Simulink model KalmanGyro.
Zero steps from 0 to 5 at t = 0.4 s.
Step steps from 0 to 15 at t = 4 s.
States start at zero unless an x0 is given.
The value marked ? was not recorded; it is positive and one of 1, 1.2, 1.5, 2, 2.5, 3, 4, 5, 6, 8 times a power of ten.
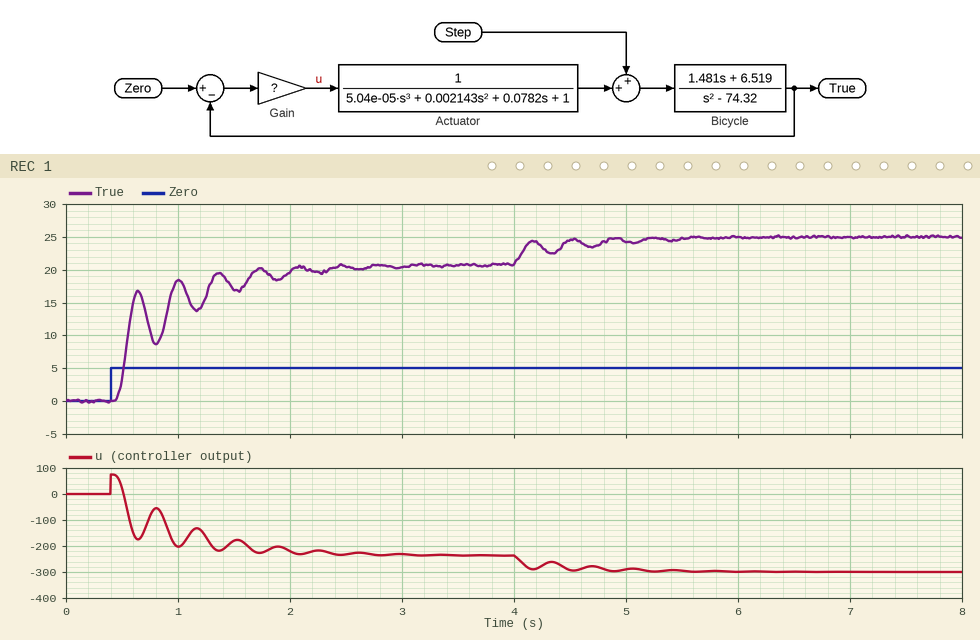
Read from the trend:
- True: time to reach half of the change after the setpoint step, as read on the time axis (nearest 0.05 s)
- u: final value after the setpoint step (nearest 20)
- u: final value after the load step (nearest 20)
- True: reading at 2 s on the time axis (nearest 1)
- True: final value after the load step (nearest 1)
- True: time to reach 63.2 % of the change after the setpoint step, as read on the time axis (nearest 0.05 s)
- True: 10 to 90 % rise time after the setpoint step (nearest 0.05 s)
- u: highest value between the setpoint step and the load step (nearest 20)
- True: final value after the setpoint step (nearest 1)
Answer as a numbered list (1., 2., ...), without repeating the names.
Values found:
1. 0.55 s
2. -240
3. -300
4. 20
5. 25
6. 0.60 s
7. 0.85 s
8. 80
9. 21
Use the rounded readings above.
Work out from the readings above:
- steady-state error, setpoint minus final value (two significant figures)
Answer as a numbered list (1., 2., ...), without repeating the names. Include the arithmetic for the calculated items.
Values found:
1. 5 - 21 = -16
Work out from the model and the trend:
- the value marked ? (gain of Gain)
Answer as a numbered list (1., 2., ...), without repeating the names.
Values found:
1. 15
